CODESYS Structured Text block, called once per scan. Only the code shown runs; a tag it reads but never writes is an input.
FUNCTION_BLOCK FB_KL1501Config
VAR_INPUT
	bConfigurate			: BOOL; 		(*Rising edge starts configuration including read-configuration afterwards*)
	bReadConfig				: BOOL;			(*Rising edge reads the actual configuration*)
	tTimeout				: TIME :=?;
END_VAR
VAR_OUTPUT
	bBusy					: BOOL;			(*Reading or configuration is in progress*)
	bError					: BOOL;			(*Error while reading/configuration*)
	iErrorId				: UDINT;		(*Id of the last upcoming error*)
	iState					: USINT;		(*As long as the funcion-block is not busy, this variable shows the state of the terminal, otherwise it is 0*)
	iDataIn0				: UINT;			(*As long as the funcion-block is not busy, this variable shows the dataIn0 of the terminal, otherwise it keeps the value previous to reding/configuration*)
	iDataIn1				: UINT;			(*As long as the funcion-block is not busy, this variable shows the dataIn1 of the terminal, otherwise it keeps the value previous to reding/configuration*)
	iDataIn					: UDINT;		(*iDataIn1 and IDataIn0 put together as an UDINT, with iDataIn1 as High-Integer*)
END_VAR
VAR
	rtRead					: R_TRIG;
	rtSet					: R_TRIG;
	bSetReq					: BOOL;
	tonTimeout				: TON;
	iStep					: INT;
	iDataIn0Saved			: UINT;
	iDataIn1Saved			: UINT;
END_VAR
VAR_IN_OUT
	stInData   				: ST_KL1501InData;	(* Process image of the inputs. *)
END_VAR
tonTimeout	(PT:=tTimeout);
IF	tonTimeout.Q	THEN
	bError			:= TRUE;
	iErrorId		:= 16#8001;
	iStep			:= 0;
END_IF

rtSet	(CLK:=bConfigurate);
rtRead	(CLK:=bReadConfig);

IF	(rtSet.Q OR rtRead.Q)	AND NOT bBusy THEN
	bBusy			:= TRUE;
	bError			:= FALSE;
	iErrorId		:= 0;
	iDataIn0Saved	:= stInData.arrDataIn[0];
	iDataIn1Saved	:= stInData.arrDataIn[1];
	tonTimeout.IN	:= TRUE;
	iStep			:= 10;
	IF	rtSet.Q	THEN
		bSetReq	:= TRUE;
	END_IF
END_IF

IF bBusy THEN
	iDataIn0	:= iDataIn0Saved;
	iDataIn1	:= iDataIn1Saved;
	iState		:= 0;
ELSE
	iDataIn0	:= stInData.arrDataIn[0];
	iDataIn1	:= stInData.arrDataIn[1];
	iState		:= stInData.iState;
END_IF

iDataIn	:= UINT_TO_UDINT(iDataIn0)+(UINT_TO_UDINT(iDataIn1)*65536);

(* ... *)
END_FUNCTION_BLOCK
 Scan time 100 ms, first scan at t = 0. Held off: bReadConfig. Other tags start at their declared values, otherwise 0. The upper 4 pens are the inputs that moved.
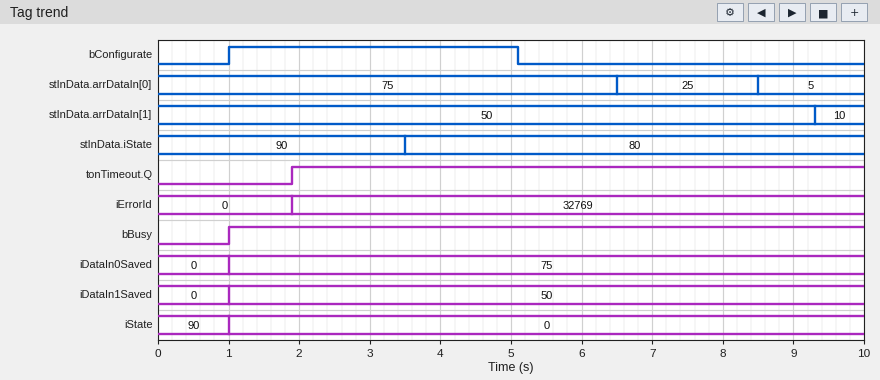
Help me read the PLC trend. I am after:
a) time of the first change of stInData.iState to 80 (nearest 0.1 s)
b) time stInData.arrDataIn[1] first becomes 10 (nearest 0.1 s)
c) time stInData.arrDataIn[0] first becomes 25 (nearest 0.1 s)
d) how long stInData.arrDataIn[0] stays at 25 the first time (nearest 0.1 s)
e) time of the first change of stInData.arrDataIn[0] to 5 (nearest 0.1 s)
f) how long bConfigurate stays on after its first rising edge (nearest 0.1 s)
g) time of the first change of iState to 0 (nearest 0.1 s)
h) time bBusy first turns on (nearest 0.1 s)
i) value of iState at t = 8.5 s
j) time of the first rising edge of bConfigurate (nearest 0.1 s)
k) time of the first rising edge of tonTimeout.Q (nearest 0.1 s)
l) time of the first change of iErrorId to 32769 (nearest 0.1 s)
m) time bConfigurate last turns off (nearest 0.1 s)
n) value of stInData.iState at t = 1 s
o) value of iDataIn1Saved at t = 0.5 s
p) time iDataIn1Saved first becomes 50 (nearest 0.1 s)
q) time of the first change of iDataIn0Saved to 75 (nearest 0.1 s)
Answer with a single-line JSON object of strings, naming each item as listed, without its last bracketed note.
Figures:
{"time of the first change of stInData.iState to 80": "3.5 s", "time stInData.arrDataIn[1] first becomes 10": "9.3 s", "time stInData.arrDataIn[0] first becomes 25": "6.5 s", "how long stInData.arrDataIn[0] stays at 25 the first time": "2.0 s", "time of the first change of stInData.arrDataIn[0] to 5": "8.5 s", "how long bConfigurate stays on after its first rising edge": "4.1 s", "time of the first change of iState to 0": "1.0 s", "time bBusy first turns on": "1.0 s", "value of iState at t = 8.5 s": "0", "time of the first rising edge of bConfigurate": "1.0 s", "time of the first rising edge of tonTimeout.Q": "1.9 s", "time of the first change of iErrorId to 32769": "1.9 s", "time bConfigurate last turns off": "5.1 s", "value of stInData.iState at t = 1 s": "90", "value of iDataIn1Saved at t = 0.5 s": "0", "time iDataIn1Saved first becomes 50": "1.0 s", "time of the first change of iDataIn0Saved to 75": "1.0 s"}
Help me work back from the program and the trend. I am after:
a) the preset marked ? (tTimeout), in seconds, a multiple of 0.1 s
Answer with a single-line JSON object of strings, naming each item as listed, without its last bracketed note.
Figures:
{"the preset marked ? (tTimeout), in seconds, a multiple of 0.1 s": "0.8 s"}
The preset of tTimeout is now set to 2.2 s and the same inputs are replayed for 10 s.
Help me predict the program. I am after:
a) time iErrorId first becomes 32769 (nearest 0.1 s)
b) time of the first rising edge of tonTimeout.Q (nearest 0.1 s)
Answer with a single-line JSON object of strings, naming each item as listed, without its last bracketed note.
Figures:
{"time iErrorId first becomes 32769": "3.3 s", "time of the first rising edge of tonTimeout.Q": "3.3 s"}
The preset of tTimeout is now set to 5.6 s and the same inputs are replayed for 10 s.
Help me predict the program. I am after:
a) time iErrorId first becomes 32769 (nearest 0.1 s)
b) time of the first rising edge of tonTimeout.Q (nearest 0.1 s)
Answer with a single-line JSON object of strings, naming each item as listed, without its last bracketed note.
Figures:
{"time iErrorId first becomes 32769": "6.7 s", "time of the first rising edge of tonTimeout.Q": "6.7 s"}
